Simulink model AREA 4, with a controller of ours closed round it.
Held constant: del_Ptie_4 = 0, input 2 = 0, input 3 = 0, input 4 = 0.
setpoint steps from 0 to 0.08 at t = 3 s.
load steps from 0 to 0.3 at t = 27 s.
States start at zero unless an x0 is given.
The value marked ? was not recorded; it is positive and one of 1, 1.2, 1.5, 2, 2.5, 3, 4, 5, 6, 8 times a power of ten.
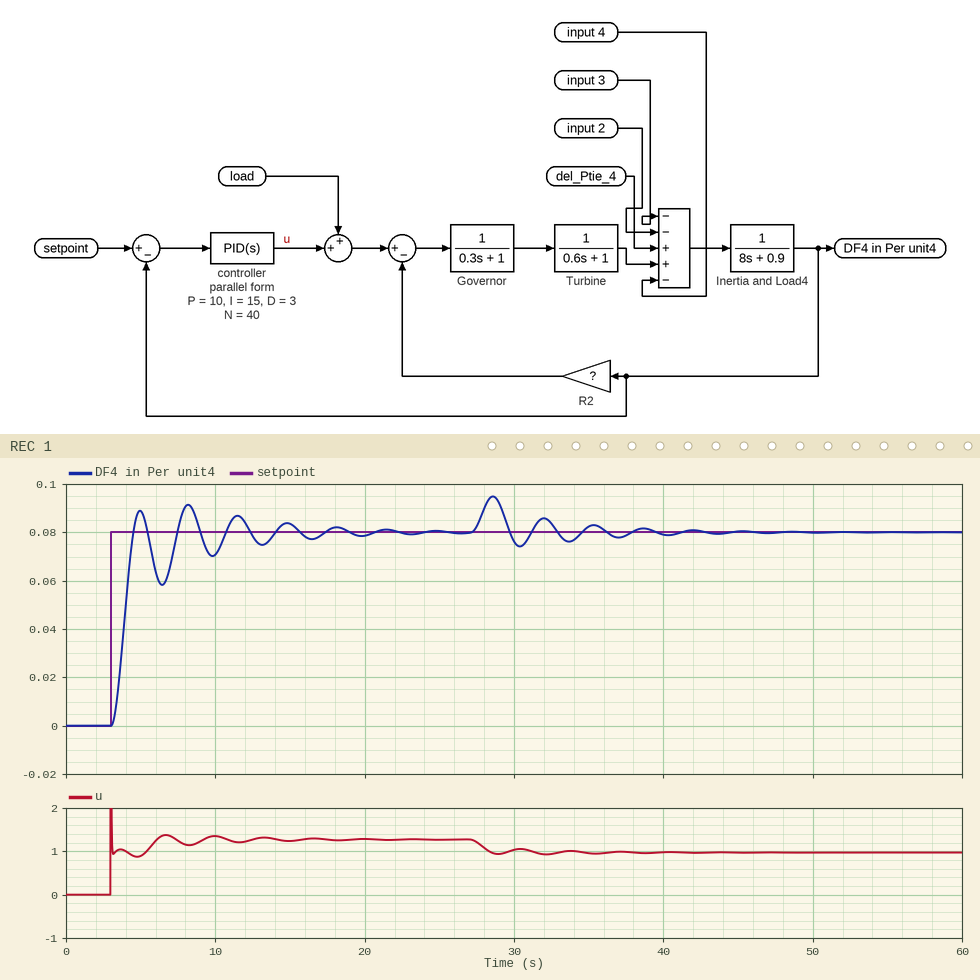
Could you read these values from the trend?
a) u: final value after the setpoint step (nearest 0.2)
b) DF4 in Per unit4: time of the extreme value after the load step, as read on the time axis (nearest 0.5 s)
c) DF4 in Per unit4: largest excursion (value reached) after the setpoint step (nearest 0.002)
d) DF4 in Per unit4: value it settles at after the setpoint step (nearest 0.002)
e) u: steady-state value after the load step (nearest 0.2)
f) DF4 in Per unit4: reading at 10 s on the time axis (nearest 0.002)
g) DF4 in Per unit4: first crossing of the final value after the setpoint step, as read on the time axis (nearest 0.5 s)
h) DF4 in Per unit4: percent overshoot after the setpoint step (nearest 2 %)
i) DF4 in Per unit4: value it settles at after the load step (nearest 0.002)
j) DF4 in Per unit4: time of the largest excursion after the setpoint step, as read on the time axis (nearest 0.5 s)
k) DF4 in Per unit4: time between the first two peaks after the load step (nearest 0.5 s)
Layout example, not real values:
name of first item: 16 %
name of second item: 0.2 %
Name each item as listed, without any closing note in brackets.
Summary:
u: final value after the setpoint step: 1.2
DF4 in Per unit4: time of the extreme value after the load step, as read on the time axis: 28.5 s
DF4 in Per unit4: largest excursion (value reached) after the setpoint step: 0.092
DF4 in Per unit4: value it settles at after the setpoint step: 0.080
u: steady-state value after the load step: 1.0
DF4 in Per unit4: reading at 10 s on the time axis: 0.070
DF4 in Per unit4: first crossing of the final value after the setpoint step, as read on the time axis: 4.5 s
DF4 in Per unit4: percent overshoot after the setpoint step: 14 %
DF4 in Per unit4: value it settles at after the load step: 0.080
DF4 in Per unit4: time of the largest excursion after the setpoint step, as read on the time axis: 8.0 s
DF4 in Per unit4: time between the first two peaks after the load step: 3.5 s
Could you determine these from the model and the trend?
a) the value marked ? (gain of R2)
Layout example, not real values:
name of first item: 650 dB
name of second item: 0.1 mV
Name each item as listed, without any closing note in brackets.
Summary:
the value marked ?: 15
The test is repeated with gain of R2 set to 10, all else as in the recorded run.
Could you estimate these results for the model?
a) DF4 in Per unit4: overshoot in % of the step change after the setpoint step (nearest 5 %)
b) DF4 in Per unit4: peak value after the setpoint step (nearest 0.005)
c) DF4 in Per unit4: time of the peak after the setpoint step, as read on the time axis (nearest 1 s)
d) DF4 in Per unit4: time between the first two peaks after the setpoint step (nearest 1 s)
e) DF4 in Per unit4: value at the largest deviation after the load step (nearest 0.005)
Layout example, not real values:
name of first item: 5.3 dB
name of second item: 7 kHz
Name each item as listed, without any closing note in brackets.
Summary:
DF4 in Per unit4: overshoot in % of the step change after the setpoint step: 30 %
DF4 in Per unit4: peak value after the setpoint step: 0.105
DF4 in Per unit4: time of the peak after the setpoint step, as read on the time axis: 5 s
DF4 in Per unit4: time between the first two peaks after the setpoint step: 4 s
DF4 in Per unit4: value at the largest deviation after the load step: 0.095
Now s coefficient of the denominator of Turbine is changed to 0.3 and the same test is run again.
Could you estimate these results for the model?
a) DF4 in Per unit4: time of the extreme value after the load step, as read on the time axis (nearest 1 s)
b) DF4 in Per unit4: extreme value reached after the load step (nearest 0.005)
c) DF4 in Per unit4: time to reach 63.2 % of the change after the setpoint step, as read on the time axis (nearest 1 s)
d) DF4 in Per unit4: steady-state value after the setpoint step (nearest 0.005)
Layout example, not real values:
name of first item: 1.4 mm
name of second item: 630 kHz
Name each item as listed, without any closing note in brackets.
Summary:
DF4 in Per unit4: time of the extreme value after the load step, as read on the time axis: 28 s
DF4 in Per unit4: extreme value reached after the load step: 0.095
DF4 in Per unit4: time to reach 63.2 % of the change after the setpoint step, as read on the time axis: 4 s
DF4 in Per unit4: steady-state value after the setpoint step: 0.080
